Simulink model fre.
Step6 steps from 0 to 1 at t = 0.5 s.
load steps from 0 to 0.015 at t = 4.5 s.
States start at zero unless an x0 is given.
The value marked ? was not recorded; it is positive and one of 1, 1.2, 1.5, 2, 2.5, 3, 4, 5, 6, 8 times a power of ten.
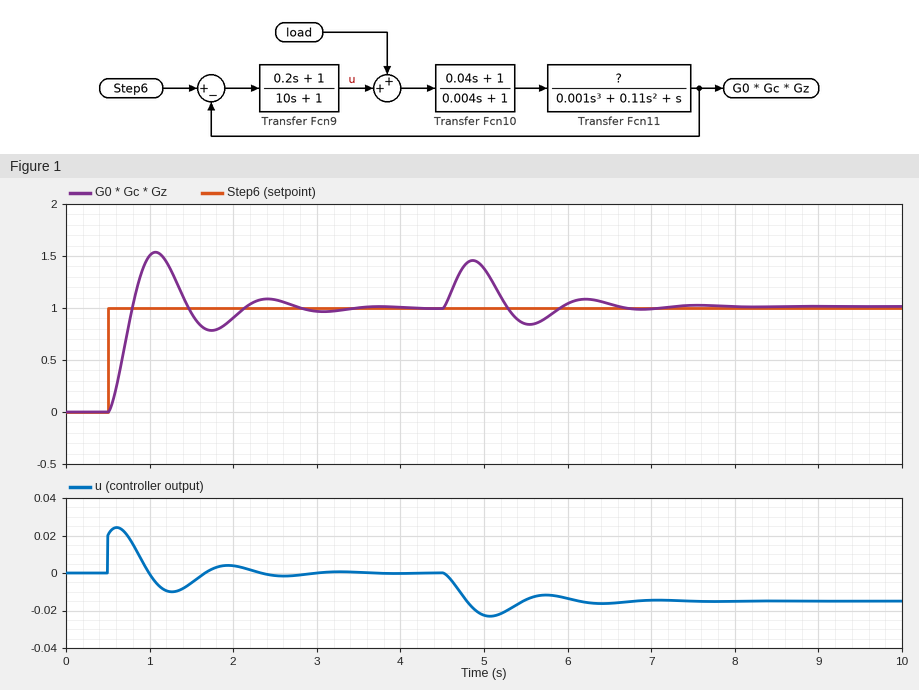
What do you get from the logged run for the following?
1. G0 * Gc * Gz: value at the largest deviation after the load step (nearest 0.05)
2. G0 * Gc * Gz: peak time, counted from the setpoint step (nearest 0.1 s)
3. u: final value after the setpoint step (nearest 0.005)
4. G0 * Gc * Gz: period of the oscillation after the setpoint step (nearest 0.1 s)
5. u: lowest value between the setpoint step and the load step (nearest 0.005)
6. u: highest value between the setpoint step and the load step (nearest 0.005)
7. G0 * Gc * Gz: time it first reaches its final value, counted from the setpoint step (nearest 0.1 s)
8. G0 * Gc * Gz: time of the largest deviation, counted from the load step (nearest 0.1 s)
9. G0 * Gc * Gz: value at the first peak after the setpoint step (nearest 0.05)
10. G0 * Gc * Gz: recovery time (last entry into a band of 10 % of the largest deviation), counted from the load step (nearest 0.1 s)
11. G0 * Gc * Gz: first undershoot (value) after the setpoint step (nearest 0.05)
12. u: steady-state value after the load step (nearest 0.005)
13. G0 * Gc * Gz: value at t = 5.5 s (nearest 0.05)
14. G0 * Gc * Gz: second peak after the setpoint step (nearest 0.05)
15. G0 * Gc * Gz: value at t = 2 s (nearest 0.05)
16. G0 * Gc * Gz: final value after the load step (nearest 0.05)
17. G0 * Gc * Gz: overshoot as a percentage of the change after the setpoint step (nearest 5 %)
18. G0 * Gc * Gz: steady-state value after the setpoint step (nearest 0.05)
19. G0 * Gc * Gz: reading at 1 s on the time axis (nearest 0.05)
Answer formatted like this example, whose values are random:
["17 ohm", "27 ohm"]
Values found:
["1.45", "0.6 s", "0.000", "1.3 s", "-0.010", "0.025", "0.3 s", "0.4 s", "1.55", "1.9 s", "0.80", "-0.015", "0.85", "1.10", "0.90", "1.00", "55 %", "1.00", "1.50"]
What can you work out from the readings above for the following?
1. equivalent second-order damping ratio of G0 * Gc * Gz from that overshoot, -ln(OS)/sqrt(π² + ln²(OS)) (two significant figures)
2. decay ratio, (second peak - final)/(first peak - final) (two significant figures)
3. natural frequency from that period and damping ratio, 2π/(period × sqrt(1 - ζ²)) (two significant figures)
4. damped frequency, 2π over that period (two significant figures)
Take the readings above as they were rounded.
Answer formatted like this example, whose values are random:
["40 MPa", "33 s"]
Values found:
["0.19", "0.18", "4.9 rad/s", "4.8 rad/s"]
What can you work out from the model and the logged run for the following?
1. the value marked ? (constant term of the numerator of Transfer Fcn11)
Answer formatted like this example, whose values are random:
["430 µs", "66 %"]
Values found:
["200"]
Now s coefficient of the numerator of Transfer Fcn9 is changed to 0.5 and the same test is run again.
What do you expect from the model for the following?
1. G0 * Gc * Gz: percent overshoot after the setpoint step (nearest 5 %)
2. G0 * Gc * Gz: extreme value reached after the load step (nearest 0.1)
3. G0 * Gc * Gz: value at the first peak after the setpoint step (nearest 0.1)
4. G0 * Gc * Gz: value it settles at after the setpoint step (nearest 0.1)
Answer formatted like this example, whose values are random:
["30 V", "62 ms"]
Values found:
["25 %", "1.3", "1.3", "1.0"]
